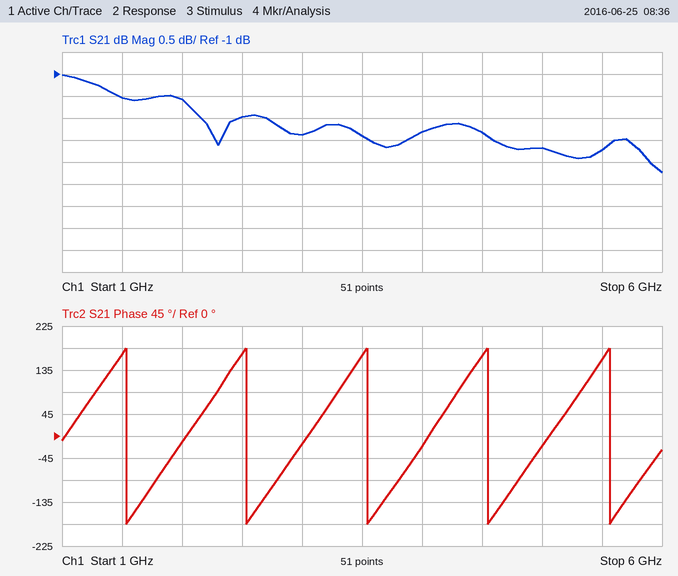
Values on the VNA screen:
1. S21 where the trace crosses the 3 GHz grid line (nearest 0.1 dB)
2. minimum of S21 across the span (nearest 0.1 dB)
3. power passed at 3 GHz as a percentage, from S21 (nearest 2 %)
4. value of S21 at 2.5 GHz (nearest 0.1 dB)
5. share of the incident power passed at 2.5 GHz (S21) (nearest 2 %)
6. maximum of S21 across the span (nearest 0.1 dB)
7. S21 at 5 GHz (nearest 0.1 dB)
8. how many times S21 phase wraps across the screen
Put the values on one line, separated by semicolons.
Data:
-2.4 dB; -3.2 dB; 58 %; -2.0 dB; 64 %; -1.0 dB; -2.7 dB; 5
